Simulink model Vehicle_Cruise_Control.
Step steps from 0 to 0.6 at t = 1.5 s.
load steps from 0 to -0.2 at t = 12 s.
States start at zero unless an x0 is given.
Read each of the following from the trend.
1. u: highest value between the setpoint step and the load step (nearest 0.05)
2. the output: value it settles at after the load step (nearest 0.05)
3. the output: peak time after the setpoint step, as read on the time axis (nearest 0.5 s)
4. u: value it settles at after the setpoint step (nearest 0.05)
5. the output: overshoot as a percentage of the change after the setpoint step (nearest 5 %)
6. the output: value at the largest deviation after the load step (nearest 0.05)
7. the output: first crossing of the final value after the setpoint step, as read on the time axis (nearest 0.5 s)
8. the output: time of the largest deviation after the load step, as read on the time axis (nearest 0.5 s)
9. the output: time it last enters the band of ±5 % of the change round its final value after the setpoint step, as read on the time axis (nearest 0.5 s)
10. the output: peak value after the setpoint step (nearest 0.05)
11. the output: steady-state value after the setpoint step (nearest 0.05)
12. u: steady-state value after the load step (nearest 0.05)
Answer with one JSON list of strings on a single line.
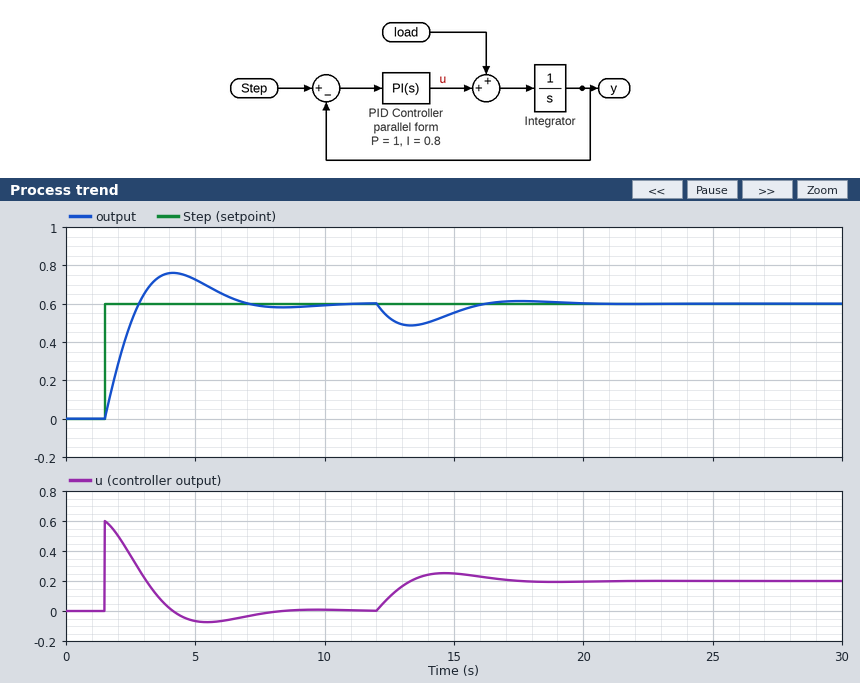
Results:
["0.60", "0.60", "4.0 s", "0.00", "25 %", "0.50", "3.0 s", "13.5 s", "6.5 s", "0.75", "0.60", "0.20"]
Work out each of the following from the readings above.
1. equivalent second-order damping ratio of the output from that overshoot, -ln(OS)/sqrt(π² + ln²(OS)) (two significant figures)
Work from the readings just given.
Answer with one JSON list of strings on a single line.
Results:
["0.40"]
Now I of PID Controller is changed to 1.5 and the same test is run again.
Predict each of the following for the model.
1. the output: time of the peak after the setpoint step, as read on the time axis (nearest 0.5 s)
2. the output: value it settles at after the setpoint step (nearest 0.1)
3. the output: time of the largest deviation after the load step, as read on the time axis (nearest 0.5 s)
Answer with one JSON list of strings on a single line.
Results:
["3.5 s", "0.6", "13.0 s"]
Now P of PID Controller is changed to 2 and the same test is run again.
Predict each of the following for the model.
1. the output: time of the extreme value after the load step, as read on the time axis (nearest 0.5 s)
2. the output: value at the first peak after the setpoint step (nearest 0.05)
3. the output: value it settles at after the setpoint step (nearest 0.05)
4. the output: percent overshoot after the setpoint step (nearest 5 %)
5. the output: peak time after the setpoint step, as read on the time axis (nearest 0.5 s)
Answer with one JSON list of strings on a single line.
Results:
["13.0 s", "0.65", "0.60", "10 %", "3.5 s"]
